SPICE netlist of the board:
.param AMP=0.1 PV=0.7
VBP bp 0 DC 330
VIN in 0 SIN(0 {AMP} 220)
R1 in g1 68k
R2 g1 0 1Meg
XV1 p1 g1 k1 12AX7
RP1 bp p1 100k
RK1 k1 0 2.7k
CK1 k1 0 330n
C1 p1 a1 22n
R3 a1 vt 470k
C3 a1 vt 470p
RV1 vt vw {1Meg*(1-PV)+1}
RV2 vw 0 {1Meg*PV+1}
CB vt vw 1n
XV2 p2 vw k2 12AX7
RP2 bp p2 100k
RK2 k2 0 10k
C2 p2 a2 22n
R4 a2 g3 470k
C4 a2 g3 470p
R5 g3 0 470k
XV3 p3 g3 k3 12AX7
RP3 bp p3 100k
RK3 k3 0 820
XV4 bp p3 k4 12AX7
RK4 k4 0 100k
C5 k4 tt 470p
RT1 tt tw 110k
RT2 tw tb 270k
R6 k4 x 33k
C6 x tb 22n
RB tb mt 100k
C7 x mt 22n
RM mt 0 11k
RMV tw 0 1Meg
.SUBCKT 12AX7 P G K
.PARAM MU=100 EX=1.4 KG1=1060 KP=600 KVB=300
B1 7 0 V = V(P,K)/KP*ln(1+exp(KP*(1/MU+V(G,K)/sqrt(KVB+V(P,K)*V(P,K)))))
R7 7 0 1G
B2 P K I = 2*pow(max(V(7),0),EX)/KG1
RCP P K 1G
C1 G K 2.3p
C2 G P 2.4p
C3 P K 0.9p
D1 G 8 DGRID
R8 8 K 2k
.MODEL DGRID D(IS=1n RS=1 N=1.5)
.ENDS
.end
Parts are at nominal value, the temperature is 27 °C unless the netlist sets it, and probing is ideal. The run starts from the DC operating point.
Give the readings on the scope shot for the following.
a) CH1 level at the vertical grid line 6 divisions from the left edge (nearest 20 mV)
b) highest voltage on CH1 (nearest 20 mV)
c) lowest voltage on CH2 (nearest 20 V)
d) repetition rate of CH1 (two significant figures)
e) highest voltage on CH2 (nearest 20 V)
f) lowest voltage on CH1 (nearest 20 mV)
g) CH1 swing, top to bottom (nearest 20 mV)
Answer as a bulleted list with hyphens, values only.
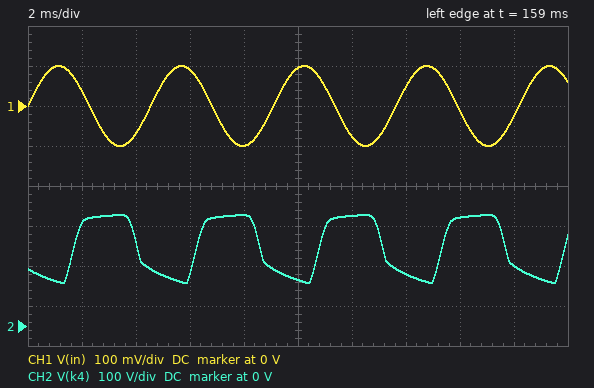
- -80 mV
- 100 mV
- 100 V
- 220 Hz
- 280 V
- -100 mV
- 200 mV
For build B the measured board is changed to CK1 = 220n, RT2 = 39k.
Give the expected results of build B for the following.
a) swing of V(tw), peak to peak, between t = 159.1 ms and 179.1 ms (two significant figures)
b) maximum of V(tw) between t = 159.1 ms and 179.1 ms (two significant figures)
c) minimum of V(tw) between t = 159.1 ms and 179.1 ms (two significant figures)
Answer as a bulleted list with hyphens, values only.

- 97 V
- 46 V
- -51 V
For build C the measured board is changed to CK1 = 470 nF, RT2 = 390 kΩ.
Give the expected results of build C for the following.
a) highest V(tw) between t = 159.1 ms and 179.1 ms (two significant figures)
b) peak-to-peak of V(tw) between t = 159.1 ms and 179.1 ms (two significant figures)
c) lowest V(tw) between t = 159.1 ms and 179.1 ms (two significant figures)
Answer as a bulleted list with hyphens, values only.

- 34 V
- 75 V
- -41 V
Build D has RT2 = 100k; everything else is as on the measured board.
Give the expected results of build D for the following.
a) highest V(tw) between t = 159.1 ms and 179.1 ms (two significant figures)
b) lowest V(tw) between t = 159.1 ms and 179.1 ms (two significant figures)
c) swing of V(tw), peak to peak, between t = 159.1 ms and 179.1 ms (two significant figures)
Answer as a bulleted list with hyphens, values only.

- 43 V
- -49 V
- 92 V
